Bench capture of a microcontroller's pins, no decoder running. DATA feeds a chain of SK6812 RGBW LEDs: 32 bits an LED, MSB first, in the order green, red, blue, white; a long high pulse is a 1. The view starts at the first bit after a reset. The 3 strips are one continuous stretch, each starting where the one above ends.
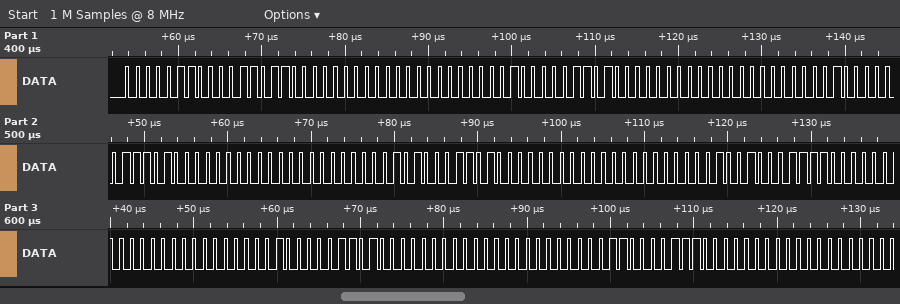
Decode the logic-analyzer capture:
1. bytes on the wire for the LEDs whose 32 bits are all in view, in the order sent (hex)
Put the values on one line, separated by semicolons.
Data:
06 1B 00 00 04 1A 00 00 08 1D 00 00 05 1A 00 00 09 1E 00 00 04 1A 00 00 06 1C 00 00
